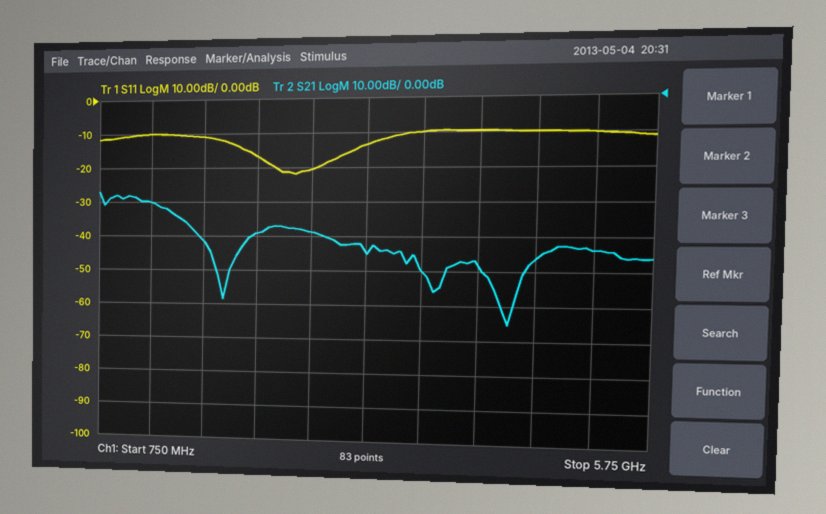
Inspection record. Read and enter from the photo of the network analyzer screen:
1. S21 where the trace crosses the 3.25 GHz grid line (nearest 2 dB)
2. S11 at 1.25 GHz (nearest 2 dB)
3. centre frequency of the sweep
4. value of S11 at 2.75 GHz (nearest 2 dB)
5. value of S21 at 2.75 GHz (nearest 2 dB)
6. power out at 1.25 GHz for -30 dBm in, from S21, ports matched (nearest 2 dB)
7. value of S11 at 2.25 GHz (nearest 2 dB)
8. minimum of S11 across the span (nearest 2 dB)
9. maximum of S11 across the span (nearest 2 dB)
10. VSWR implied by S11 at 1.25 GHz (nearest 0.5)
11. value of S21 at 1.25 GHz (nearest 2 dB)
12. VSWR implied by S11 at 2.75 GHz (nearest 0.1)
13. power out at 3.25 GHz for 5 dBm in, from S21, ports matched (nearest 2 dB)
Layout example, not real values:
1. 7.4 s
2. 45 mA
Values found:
1. -44 dB
2. -10 dB
3. 3.25 GHz
4. -20 dB
5. -38 dB
6. -60 dBm
7. -16 dB
8. -22 dB
9. -10 dB
10. 2.0
11. -30 dB
12. 1.2
13. -40 dBm
